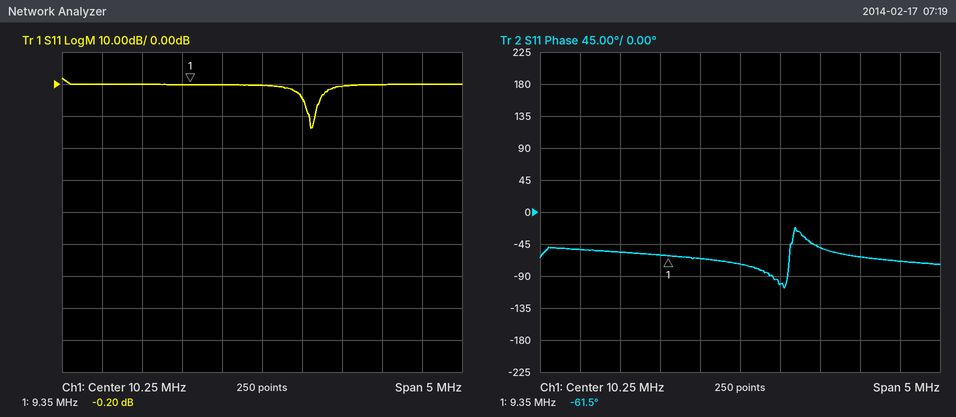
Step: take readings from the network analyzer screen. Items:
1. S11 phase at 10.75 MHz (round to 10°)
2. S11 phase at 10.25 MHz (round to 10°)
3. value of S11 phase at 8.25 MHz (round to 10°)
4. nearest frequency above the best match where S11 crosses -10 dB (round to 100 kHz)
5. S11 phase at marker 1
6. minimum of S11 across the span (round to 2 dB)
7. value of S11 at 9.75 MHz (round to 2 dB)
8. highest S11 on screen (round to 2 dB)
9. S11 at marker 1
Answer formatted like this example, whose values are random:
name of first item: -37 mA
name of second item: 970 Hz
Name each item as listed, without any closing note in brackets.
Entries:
S11 phase at 10.75 MHz: -100°
S11 phase at 10.25 MHz: -70°
value of S11 phase at 8.25 MHz: -50°
nearest frequency above the best match where S11 crosses -10 dB: 10.9 MHz
S11 phase at marker 1: -61.5°
minimum of S11 across the span: -14 dB
value of S11 at 9.75 MHz: 0 dB
highest S11 on screen: 2 dB
S11 at marker 1: -0.20 dB
